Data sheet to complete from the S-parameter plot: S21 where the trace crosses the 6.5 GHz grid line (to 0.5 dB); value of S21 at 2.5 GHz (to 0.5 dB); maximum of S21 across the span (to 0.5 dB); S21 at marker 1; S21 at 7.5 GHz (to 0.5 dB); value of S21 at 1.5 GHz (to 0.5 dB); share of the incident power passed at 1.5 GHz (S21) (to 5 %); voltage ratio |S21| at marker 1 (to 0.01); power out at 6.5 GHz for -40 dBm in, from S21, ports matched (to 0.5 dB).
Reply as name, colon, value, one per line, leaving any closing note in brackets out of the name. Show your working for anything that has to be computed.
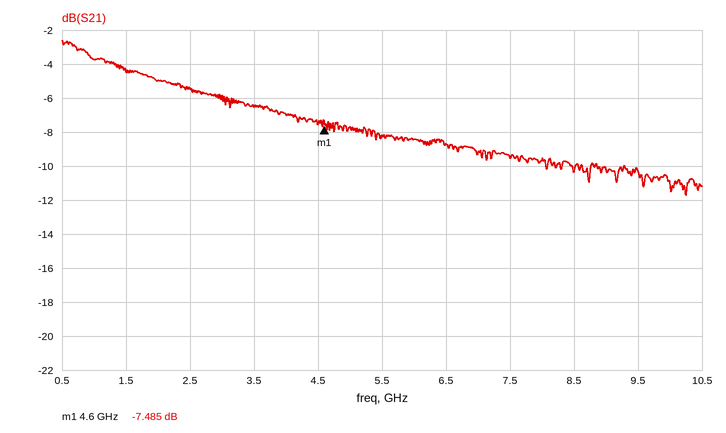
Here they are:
S21 where the trace crosses the 6.5 GHz grid line: -8.5 dB
value of S21 at 2.5 GHz: -5.5 dB
maximum of S21 across the span: -2.5 dB
S21 at marker 1: -7.485 dB
S21 at 7.5 GHz: -9.5 dB
value of S21 at 1.5 GHz: -4.5 dB
share of the incident power passed at 1.5 GHz (S21): 10^(-4.5/10) ≈ 35 %
voltage ratio |S21| at marker 1: 10^(-7.485/20) ≈ 0.42
power out at 6.5 GHz for -40 dBm in, from S21, ports matched: -40 dBm + (-8.5 dB) = -48.5 dBm
